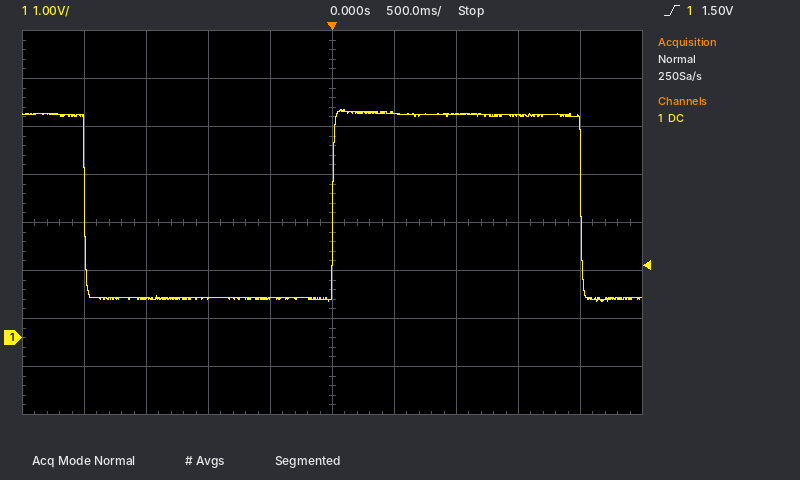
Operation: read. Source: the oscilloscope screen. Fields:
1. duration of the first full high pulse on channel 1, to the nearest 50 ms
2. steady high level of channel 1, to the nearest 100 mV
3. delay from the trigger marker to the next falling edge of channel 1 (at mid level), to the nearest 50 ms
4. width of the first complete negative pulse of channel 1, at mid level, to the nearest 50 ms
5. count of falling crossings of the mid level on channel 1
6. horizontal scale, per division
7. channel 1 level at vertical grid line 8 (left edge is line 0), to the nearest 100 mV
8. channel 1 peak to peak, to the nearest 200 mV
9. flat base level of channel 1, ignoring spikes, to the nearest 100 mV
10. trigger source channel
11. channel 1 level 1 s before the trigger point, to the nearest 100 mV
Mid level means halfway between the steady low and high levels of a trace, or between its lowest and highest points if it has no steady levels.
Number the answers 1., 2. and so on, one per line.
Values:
1. 2.00 s
2. 4.6 V
3. 2.00 s
4. 2.00 s
5. 2
6. 500 ms
7. 4.6 V
8. 4.0 V
9. 800 mV
10. channel 1
11. 800 mV
